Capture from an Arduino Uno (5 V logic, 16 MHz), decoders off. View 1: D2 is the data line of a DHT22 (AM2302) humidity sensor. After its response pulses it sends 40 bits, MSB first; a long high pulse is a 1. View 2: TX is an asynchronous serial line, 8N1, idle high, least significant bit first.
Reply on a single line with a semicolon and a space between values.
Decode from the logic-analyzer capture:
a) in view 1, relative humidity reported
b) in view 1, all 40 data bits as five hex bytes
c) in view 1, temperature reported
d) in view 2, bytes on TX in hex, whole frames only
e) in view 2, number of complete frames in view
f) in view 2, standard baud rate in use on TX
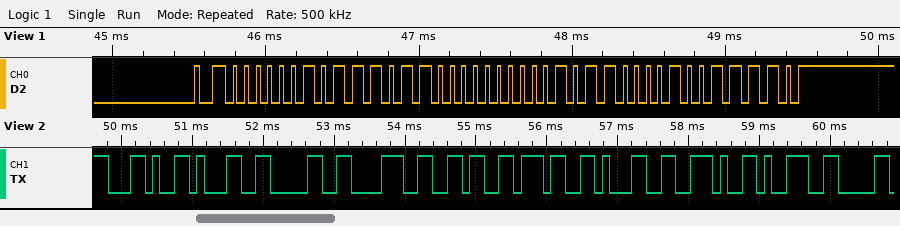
74.8 %; 02 EC 00 B0 9E; 17.6 °C; 2C 31 30 38 36 37 31 2E 39; 9; 9600 baud
